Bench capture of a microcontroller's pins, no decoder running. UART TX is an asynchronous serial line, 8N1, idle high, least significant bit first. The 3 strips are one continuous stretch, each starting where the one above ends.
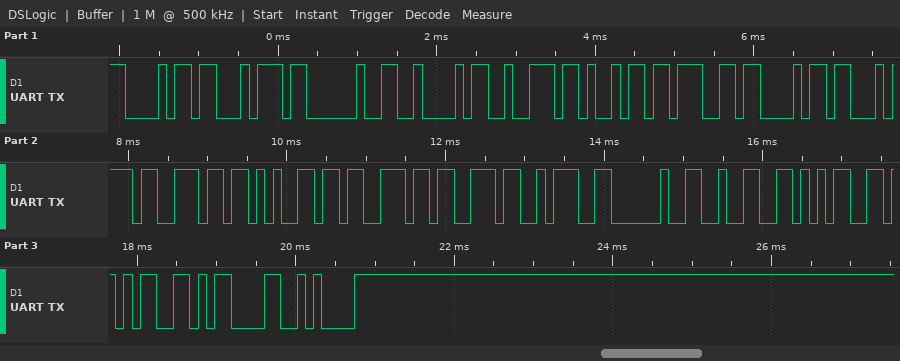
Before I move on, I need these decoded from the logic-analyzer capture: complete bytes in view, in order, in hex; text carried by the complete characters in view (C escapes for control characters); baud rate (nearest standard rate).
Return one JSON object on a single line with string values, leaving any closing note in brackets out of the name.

{"complete bytes in view, in order, in hex": "68 74 20 42 72 69 67 68 74 6E 65 73 73 3A 20 32 35 35 0D 0A", "text carried by the complete characters in view": "\"ht Brightness: 255\\r\\n\"", "baud rate": "9600 baud"}
